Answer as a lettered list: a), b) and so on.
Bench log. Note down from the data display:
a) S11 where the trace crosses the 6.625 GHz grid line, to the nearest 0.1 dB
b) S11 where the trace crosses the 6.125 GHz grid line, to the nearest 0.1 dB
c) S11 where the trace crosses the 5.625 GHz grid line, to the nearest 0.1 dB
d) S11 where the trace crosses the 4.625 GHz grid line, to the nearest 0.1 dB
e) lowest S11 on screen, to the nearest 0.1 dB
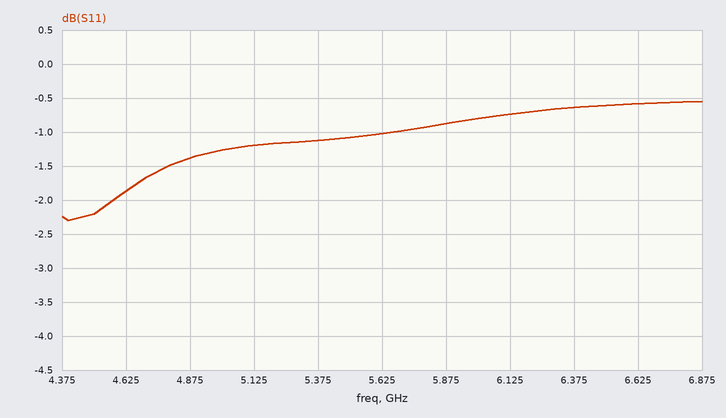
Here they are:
a) -0.6 dB
b) -0.7 dB
c) -1.0 dB
d) -1.9 dB
e) -2.3 dB
